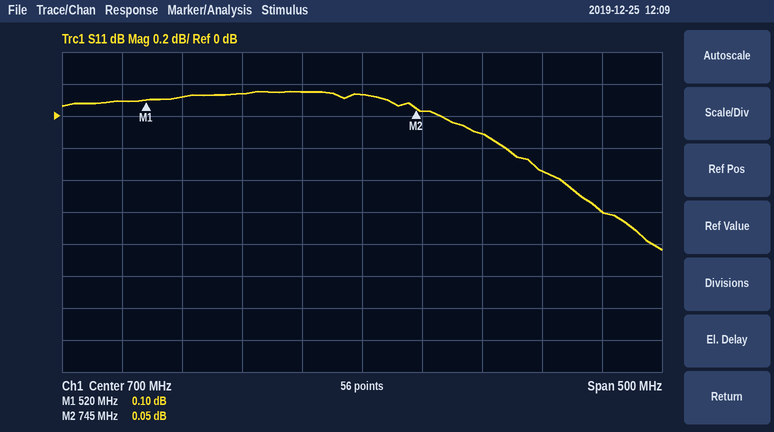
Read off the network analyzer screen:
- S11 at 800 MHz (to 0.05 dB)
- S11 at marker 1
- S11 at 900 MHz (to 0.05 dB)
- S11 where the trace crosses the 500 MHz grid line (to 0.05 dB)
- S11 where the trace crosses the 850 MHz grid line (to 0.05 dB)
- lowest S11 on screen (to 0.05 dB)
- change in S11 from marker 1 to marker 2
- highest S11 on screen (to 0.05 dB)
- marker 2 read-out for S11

-0.10 dB
0.10 dB
-0.60 dB
0.10 dB
-0.35 dB
-0.85 dB
-0.05 dB
0.15 dB
0.05 dB
